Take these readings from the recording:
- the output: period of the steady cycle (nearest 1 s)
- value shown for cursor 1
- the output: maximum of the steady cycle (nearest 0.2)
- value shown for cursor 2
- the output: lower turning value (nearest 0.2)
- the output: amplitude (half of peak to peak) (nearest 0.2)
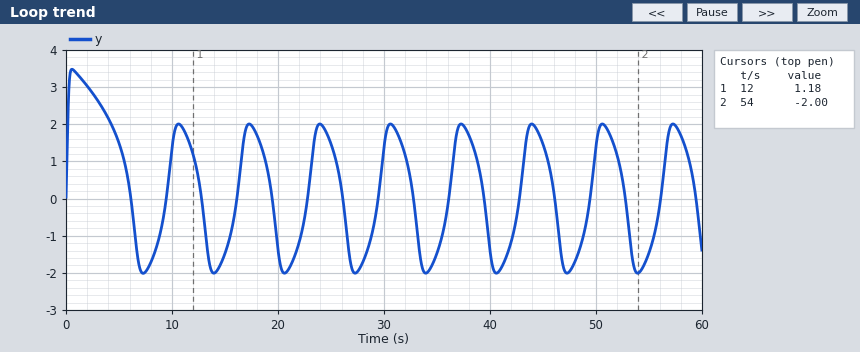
7 s
1.18
2.0
-2.00
-2.0
2.0
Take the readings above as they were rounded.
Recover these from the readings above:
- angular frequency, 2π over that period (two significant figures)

0.90 rad/s
